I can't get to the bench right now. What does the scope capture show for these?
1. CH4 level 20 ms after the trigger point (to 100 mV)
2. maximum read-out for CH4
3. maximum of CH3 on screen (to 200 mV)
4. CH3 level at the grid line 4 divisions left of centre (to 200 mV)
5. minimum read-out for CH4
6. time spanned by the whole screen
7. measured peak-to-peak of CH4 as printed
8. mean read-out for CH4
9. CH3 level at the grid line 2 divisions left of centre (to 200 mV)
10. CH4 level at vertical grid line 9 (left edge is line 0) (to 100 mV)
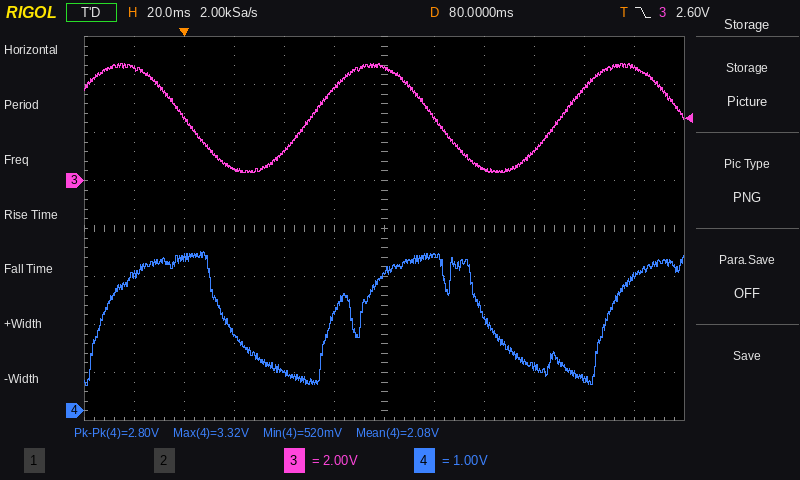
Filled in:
1.6 V
3.32 V
4.8 V
2.6 V
520 mV
240 ms
2.80 V
2.08 V
1.2 V
900 mV
